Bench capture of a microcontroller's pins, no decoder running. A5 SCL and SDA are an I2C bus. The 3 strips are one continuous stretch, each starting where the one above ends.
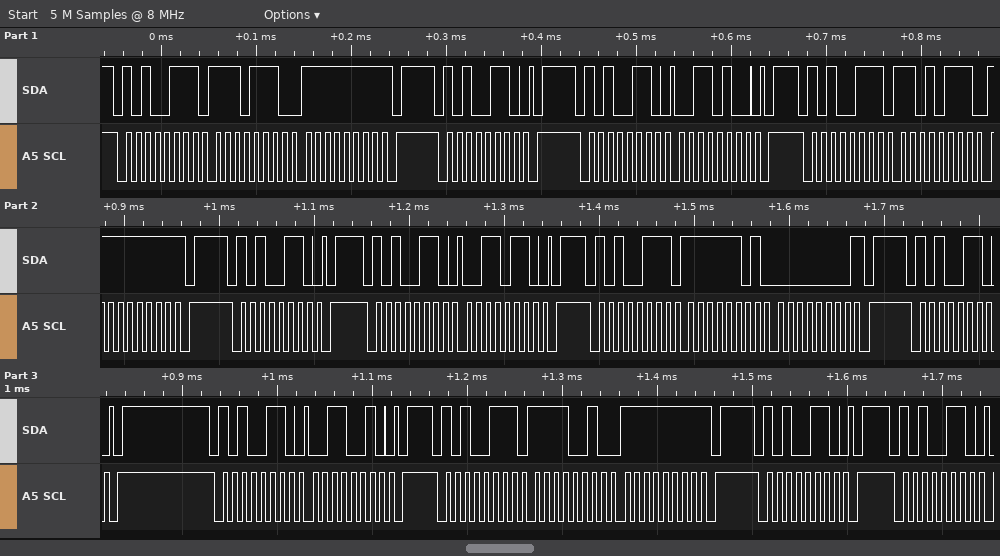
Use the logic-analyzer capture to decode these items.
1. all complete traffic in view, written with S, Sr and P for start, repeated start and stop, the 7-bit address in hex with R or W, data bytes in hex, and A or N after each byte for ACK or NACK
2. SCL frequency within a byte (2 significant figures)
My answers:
S 53R A EE A FF N P S 53W A P S 53W A 34 A P S 53R A D7 A FF N P S 53W A P S 53W A 36 A P S 53R A FD A 00 N P S 53W A P S 53W A 32 A P S 53R A F2 A FF N P S 53W A P S 53W A
100 kHz
